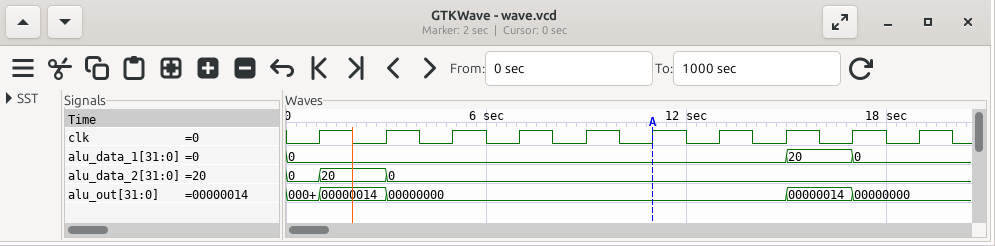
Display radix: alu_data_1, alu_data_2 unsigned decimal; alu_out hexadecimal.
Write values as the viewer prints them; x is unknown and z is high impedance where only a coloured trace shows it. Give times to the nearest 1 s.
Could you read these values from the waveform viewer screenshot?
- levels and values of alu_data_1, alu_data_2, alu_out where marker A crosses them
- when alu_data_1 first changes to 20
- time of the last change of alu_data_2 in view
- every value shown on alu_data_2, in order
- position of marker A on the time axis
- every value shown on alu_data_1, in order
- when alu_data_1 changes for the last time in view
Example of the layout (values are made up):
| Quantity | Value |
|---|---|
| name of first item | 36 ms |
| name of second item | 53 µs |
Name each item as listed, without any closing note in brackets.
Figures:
| Quantity | Value |
|---|---|
| levels and values of alu_data_1, alu_data_2, alu_out where marker A crosses them | alu_data_1=0, alu_data_2=0, alu_out=00000000 |
| when alu_data_1 first changes to 20 | 15 s |
| time of the last change of alu_data_2 in view | 3 s |
| every value shown on alu_data_2, in order | 0, 20, 0 |
| position of marker A on the time axis | 11 s |
| every value shown on alu_data_1, in order | 0, 20, 0 |
| when alu_data_1 changes for the last time in view | 17 s |
